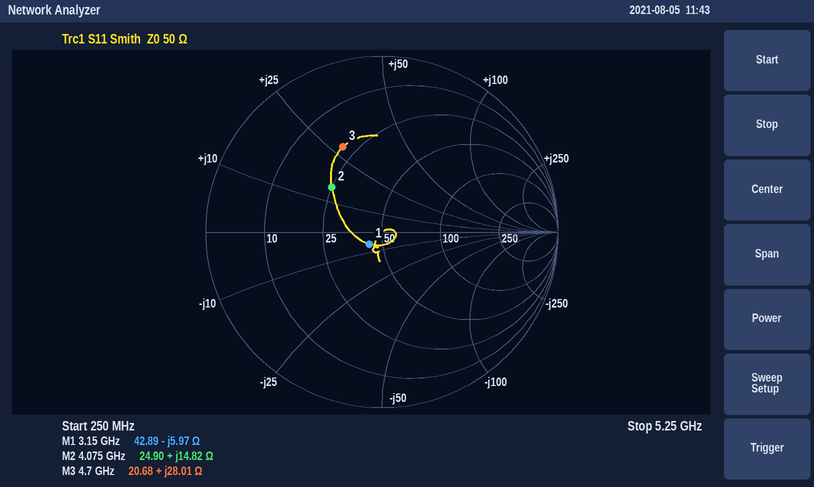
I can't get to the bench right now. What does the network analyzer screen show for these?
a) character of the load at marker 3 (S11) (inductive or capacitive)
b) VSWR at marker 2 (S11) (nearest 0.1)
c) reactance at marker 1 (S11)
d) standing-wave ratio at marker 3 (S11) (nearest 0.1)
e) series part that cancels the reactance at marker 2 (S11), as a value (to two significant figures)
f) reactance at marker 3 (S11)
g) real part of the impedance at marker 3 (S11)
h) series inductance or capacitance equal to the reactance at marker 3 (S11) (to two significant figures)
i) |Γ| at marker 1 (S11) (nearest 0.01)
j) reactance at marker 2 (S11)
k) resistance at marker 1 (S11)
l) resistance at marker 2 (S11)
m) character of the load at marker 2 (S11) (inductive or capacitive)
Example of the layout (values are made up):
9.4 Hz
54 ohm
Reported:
inductive
2.2
-5.97 Ω
3.3
2.6 pF
+28.01 Ω
20.68 Ω
950 pH
0.10
+14.82 Ω
42.89 Ω
24.90 Ω
inductive
